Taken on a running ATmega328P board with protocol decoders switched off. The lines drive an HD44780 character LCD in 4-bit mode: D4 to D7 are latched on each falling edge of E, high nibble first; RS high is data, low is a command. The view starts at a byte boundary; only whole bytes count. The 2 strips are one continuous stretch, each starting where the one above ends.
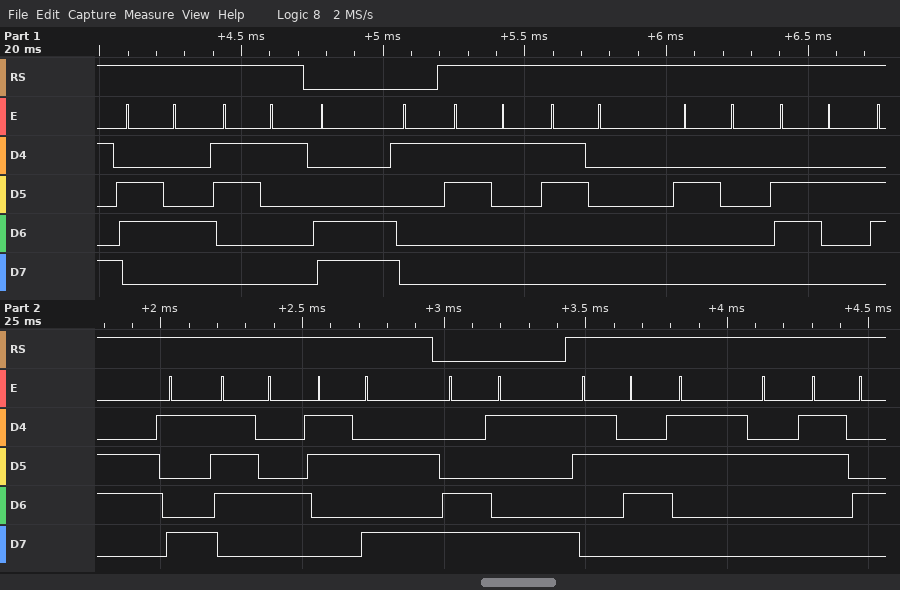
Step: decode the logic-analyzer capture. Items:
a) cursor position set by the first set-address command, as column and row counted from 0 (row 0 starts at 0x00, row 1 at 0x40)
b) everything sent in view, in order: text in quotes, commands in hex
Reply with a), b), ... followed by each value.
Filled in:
a) column 1, row 1
b) "d1" 0xC1 "10 bit:" 0xC9 "624"
